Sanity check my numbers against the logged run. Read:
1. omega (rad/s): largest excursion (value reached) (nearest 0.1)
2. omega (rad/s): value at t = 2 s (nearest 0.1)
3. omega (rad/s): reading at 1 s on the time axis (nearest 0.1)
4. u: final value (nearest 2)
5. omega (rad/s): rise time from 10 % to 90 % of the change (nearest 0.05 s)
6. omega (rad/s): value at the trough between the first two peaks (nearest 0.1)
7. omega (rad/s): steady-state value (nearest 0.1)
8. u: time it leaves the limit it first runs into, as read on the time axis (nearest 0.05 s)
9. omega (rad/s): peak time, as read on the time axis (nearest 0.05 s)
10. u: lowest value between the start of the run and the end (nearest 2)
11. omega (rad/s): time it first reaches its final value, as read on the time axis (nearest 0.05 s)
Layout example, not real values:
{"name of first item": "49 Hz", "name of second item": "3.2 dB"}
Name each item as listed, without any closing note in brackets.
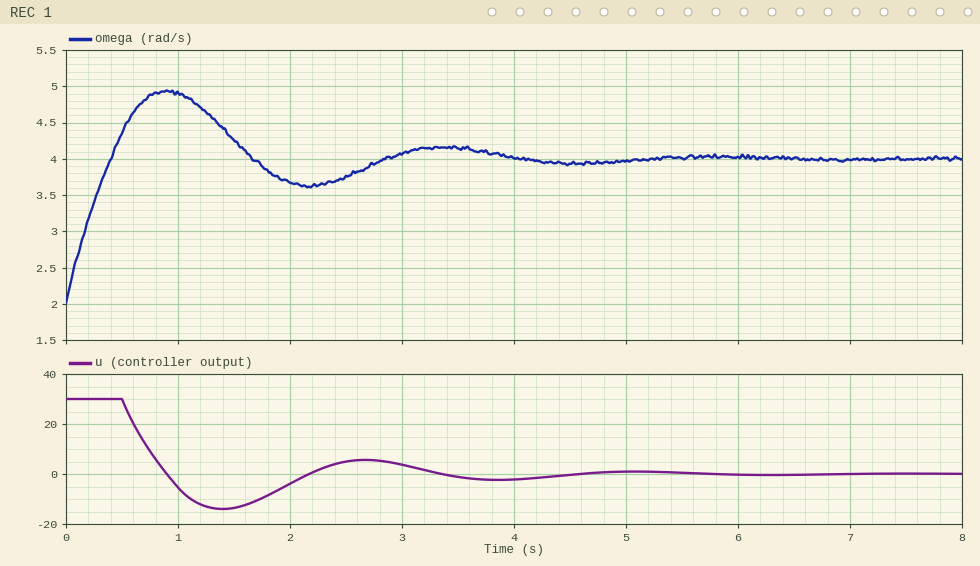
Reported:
{"omega (rad/s): largest excursion (value reached)": "4.9", "omega (rad/s): value at t = 2 s": "3.7", "omega (rad/s): reading at 1 s on the time axis": "4.9", "u: final value": "0", "omega (rad/s): rise time from 10 % to 90 % of the change": "0.30 s", "omega (rad/s): value at the trough between the first two peaks": "3.6", "omega (rad/s): steady-state value": "4.0", "u: time it leaves the limit it first runs into, as read on the time axis": "0.50 s", "omega (rad/s): peak time, as read on the time axis": "0.90 s", "u: lowest value between the start of the run and the end": "-14", "omega (rad/s): time it first reaches its final value, as read on the time axis": "0.40 s"}
